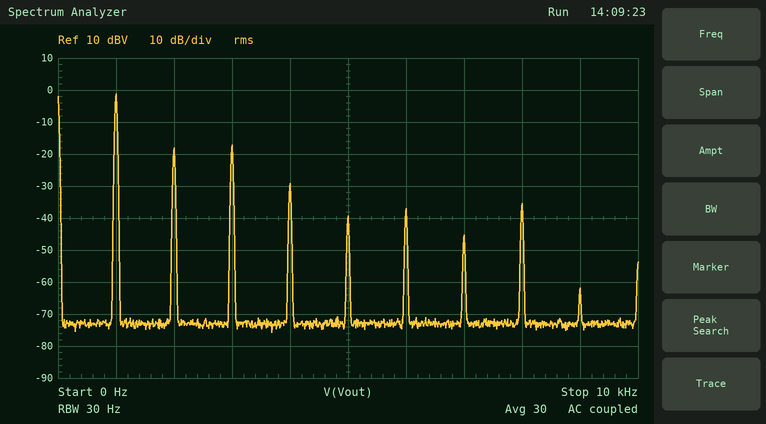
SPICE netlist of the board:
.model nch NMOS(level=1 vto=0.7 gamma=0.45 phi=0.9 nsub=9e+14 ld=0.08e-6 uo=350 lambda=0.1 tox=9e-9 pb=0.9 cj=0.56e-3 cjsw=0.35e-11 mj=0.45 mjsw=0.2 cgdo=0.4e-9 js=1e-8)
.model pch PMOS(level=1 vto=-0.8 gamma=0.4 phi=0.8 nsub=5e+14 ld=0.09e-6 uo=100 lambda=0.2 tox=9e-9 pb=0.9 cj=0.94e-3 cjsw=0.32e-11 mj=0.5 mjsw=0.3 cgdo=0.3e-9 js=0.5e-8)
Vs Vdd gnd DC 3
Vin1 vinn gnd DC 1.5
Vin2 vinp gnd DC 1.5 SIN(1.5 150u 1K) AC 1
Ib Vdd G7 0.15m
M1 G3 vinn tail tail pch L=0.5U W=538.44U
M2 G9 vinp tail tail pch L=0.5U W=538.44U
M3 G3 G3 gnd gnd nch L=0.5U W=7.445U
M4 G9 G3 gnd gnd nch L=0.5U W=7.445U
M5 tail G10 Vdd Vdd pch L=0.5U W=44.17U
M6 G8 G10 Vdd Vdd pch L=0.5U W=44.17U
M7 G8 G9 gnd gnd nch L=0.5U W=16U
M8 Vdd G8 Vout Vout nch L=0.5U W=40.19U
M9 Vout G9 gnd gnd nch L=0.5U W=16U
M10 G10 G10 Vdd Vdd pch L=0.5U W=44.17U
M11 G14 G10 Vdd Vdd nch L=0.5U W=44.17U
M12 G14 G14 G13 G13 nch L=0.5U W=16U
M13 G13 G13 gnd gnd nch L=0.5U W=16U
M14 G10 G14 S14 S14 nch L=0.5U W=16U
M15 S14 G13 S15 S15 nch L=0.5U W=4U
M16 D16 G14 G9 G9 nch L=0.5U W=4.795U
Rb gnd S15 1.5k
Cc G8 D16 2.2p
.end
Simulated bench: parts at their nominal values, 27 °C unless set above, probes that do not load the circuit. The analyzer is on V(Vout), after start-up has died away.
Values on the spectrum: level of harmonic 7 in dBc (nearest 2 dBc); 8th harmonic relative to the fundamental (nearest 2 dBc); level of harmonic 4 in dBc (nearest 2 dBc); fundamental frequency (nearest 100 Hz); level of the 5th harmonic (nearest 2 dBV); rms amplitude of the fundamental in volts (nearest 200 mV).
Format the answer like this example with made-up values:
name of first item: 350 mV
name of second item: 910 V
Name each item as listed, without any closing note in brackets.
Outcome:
level of harmonic 7 in dBc: -44 dBc
8th harmonic relative to the fundamental: -34 dBc
level of harmonic 4 in dBc: -28 dBc
fundamental frequency: 1.0 kHz
level of the 5th harmonic: -40 dBV
rms amplitude of the fundamental in volts: 800 mV
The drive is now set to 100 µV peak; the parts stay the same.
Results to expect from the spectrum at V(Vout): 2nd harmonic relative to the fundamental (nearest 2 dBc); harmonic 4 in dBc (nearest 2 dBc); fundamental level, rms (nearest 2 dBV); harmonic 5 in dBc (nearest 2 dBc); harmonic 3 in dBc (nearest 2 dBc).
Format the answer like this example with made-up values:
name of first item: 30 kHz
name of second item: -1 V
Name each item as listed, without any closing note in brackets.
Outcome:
2nd harmonic relative to the fundamental: -18 dBc
harmonic 4 in dBc: -32 dBc
fundamental level, rms: -2 dBV
harmonic 5 in dBc: -54 dBc
harmonic 3 in dBc: -24 dBc
